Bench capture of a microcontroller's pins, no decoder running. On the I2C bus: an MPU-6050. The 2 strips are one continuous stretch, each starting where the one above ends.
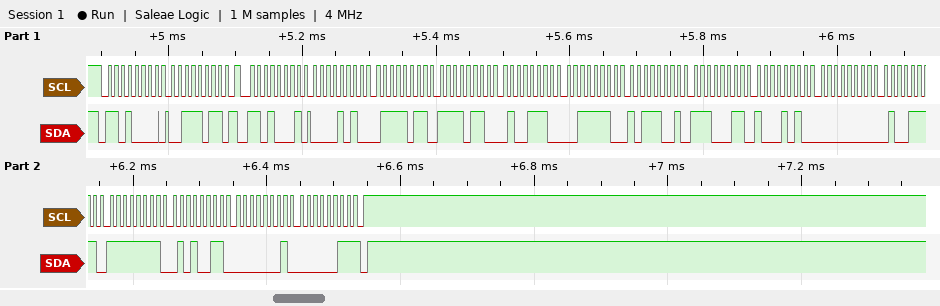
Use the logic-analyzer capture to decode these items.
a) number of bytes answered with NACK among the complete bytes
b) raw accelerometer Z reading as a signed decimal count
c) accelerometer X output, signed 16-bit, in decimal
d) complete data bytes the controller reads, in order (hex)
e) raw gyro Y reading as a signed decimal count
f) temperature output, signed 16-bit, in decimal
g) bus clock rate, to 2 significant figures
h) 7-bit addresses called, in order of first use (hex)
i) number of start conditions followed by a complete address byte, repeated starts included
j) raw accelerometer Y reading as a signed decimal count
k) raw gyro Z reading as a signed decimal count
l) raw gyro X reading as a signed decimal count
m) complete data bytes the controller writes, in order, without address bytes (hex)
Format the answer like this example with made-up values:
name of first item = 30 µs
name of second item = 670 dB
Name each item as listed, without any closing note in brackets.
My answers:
number of bytes answered with NACK among the complete bytes = 1
raw accelerometer Z reading as a signed decimal count = 16057
accelerometer X output, signed 16-bit, in decimal = 2683
complete data bytes the controller reads, in order = 0A 7B F6 4E 3E B9 E3 8A 00 4F FF 53 01 03
raw gyro Y reading as a signed decimal count = -173
temperature output, signed 16-bit, in decimal = -7286
bus clock rate, to 2 significant figures = 100 kHz
7-bit addresses called, in order of first use = 0x68
number of start conditions followed by a complete address byte, repeated starts included = 2
raw accelerometer Y reading as a signed decimal count = -2482
raw gyro Z reading as a signed decimal count = 259
raw gyro X reading as a signed decimal count = 79
complete data bytes the controller writes, in order, without address bytes = 3B
